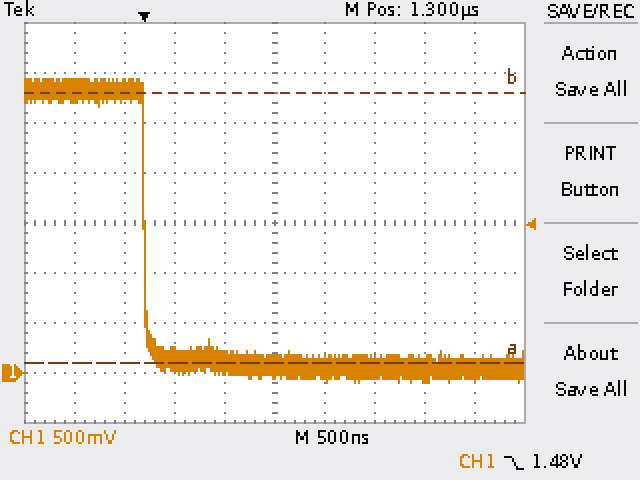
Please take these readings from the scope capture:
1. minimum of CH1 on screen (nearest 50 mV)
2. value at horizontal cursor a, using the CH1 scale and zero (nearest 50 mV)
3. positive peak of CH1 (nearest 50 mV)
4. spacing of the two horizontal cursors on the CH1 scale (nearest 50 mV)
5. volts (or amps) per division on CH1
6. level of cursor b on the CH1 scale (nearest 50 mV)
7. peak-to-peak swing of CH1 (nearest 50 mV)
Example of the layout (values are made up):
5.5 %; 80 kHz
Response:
-100 mV; 100 mV; 2.95 V; 2.70 V; 500 mV; 2.80 V; 3.05 V
